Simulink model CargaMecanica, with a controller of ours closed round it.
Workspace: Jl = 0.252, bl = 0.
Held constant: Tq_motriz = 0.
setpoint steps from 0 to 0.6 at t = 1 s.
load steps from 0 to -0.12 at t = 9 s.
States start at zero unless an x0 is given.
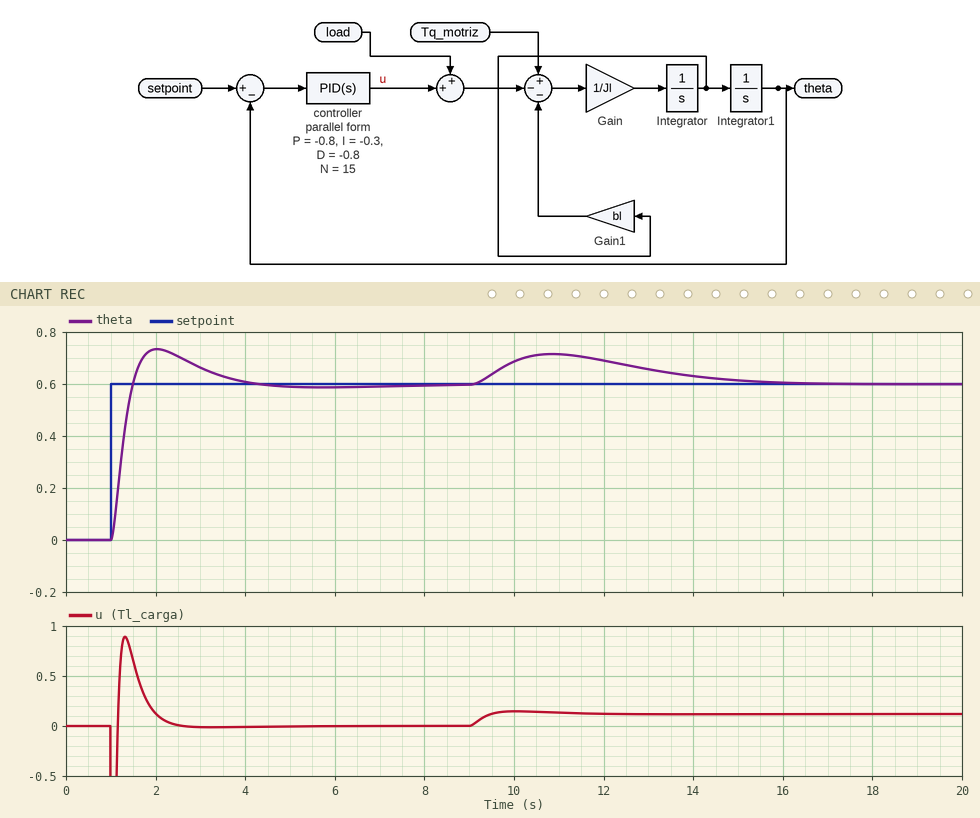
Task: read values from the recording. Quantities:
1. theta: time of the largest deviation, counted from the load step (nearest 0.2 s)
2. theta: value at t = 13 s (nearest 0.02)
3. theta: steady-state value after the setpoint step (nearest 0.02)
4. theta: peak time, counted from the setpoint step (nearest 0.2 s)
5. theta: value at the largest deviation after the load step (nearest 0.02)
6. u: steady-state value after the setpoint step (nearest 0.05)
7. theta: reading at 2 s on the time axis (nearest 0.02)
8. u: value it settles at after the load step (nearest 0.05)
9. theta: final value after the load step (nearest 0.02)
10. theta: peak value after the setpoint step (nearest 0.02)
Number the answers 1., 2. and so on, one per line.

1. 1.8 s
2. 0.66
3. 0.60
4. 1.0 s
5. 0.72
6. 0.00
7. 0.74
8. 0.10
9. 0.60
10. 0.74
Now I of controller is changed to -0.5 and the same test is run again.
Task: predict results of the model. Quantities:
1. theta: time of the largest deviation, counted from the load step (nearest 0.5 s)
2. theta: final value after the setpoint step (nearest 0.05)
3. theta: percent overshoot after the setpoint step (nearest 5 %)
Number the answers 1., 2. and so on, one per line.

1. 1.5 s
2. 0.60
3. 25 %
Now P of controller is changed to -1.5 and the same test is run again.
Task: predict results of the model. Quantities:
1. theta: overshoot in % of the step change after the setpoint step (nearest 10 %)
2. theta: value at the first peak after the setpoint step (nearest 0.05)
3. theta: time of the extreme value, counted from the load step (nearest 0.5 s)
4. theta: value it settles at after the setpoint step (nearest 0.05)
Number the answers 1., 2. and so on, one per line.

1. 30 %
2. 0.80
3. 1.5 s
4. 0.60
